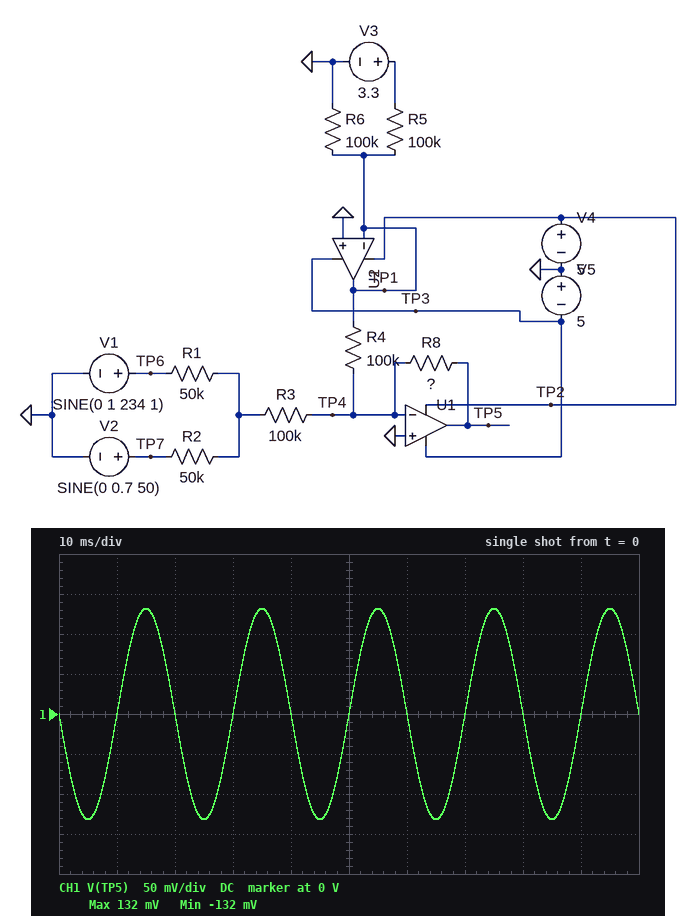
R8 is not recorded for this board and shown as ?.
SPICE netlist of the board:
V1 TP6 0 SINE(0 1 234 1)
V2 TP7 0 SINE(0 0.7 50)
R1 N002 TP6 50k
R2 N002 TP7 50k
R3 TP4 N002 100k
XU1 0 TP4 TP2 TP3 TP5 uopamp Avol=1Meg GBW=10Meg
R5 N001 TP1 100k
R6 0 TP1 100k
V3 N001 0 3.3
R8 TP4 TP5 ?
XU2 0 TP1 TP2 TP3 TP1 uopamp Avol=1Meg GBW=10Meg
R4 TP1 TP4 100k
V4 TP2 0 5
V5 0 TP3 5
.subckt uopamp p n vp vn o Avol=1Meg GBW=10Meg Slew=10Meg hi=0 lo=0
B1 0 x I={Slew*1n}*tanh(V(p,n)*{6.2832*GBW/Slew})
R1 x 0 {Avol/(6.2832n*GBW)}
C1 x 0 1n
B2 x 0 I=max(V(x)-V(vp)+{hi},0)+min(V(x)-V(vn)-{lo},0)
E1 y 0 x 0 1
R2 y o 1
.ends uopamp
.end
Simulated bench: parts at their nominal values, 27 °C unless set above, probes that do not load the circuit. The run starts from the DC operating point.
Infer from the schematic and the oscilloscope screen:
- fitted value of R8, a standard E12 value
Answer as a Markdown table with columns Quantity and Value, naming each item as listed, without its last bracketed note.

| Quantity | Value |
|---|---|
| fitted value of R8, a standard E12 value | 47 kΩ |
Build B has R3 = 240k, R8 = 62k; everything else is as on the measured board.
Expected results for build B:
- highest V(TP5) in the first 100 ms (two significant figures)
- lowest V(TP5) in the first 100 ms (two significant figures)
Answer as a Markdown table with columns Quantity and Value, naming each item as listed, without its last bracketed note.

| Quantity | Value |
|---|---|
| highest V(TP5) in the first 100 ms | 82 mV |
| lowest V(TP5) in the first 100 ms | -82 mV |
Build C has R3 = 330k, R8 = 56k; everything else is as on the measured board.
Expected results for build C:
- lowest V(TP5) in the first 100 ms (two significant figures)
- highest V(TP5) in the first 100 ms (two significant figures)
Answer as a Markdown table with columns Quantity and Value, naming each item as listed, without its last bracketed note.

| Quantity | Value |
|---|---|
| lowest V(TP5) in the first 100 ms | -55 mV |
| highest V(TP5) in the first 100 ms | 55 mV |
